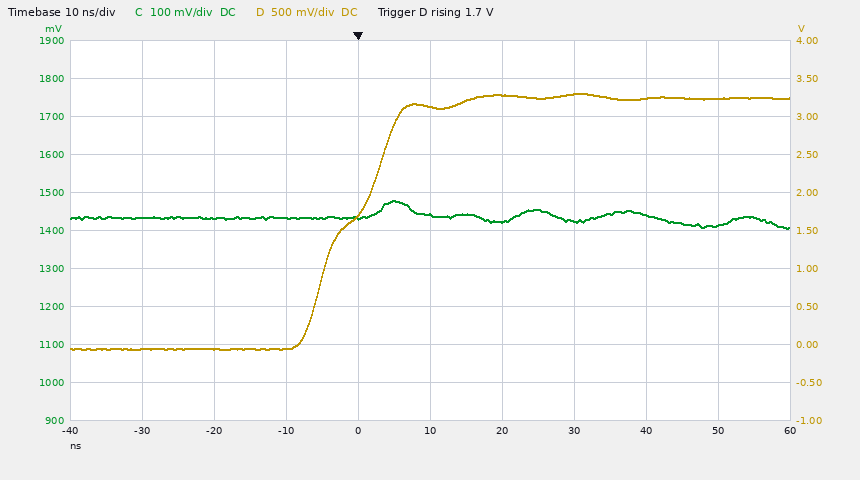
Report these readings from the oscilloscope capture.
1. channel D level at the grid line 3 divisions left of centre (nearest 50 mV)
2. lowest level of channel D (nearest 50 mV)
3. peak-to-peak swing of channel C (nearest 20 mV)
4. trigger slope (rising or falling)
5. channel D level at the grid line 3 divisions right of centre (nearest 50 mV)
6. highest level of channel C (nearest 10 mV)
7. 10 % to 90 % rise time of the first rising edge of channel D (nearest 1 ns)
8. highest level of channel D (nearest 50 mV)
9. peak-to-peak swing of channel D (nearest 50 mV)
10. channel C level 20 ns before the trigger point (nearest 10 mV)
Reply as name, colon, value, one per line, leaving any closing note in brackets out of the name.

channel D level at the grid line 3 divisions left of centre: -50 mV
lowest level of channel D: -50 mV
peak-to-peak swing of channel C: 80 mV
trigger slope: rising
channel D level at the grid line 3 divisions right of centre: 3.25 V
highest level of channel C: 1.48 V
10 % to 90 % rise time of the first rising edge of channel D: 12 ns
highest level of channel D: 3.30 V
peak-to-peak swing of channel D: 3.35 V
channel C level 20 ns before the trigger point: 1.43 V
